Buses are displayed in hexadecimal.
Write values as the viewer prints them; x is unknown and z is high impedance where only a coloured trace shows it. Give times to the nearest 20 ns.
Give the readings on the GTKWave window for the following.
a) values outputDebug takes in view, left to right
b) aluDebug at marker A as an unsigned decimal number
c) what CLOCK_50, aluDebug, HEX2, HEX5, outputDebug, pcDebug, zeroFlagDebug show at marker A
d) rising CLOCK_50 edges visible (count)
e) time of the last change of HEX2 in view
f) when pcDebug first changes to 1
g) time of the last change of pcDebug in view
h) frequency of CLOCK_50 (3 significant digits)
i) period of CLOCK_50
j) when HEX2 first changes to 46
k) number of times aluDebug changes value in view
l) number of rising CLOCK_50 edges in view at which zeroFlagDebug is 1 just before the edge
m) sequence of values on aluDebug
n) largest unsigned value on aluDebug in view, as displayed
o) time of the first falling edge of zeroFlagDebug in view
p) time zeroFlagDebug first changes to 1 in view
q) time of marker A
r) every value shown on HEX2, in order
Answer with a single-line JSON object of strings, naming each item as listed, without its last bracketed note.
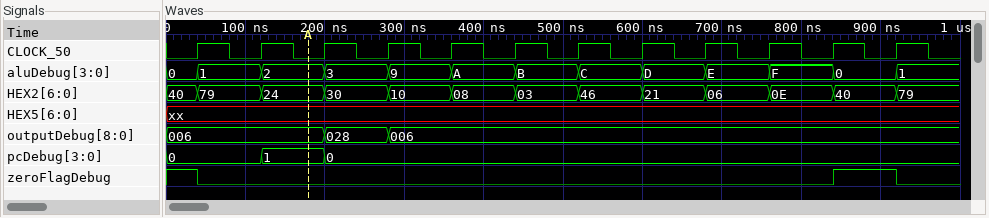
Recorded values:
{"values outputDebug takes in view, left to right": "006, 028, 006", "aluDebug at marker A as an unsigned decimal number": "2", "what CLOCK_50, aluDebug, HEX2, HEX5, outputDebug, pcDebug, zeroFlagDebug show at marker A": "CLOCK_50=0, aluDebug=2, HEX2=24, HEX5=xx, outputDebug=006, pcDebug=1, zeroFlagDebug=0", "rising CLOCK_50 edges visible": "12", "time of the last change of HEX2 in view": "920 ns", "when pcDebug first changes to 1": "120 ns", "time of the last change of pcDebug in view": "200 ns", "frequency of CLOCK_50": "12.5 MHz", "period of CLOCK_50": "80 ns", "when HEX2 first changes to 46": "520 ns", "number of times aluDebug changes value in view": "12", "number of rising CLOCK_50 edges in view at which zeroFlagDebug is 1 just before the edge": "2", "sequence of values on aluDebug": "0, 1, 2, 3, 9, A, B, C, D, E, F, 0, 1", "largest unsigned value on aluDebug in view, as displayed": "F", "time of the first falling edge of zeroFlagDebug in view": "40 ns", "time zeroFlagDebug first changes to 1 in view": "840 ns", "time of marker A": "180 ns", "every value shown on HEX2, in order": "40, 79, 24, 30, 10, 08, 03, 46, 21, 06, 0E, 40, 79"}
